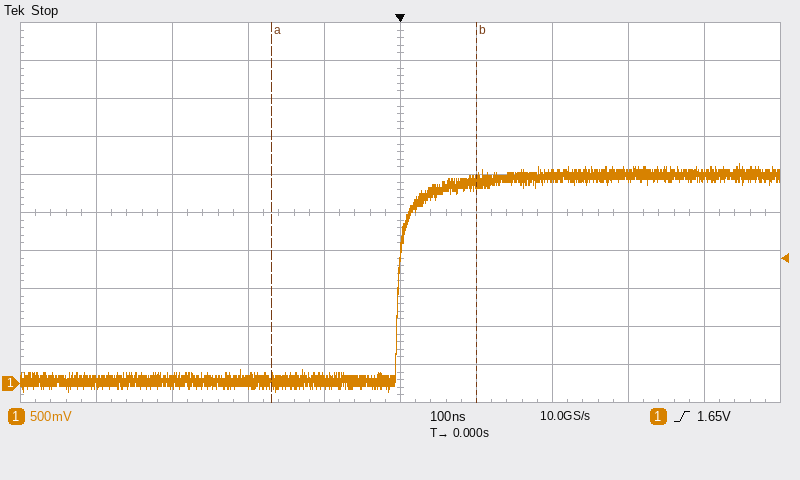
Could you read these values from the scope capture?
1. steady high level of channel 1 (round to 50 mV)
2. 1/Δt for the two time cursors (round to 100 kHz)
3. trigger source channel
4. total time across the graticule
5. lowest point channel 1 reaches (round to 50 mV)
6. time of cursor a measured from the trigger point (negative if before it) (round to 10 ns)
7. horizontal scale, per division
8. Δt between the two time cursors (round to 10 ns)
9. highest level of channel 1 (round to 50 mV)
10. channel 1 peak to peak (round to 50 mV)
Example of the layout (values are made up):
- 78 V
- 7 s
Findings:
- 2.75 V
- 3.7 MHz
- channel 1
- 1 µs
- -100 mV
- -170 ns
- 100 ns
- 270 ns
- 2.90 V
- 3.00 V
